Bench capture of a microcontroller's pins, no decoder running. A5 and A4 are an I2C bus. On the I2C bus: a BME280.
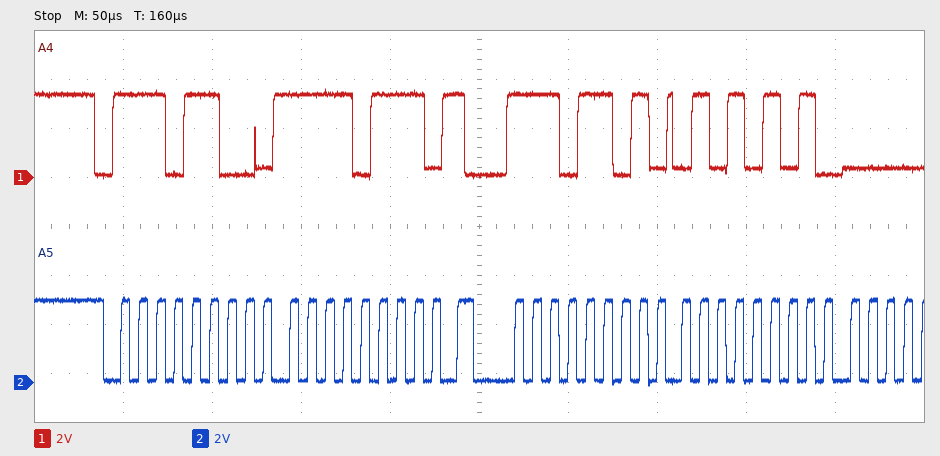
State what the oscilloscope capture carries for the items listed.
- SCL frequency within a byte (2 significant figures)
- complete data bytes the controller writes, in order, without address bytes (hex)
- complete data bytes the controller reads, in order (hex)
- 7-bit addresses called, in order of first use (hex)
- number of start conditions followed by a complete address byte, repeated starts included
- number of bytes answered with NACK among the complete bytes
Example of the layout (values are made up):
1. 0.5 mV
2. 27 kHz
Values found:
1. 100 kHz
2. F7
3. 55
4. 0x76
5. 2
6. 0
